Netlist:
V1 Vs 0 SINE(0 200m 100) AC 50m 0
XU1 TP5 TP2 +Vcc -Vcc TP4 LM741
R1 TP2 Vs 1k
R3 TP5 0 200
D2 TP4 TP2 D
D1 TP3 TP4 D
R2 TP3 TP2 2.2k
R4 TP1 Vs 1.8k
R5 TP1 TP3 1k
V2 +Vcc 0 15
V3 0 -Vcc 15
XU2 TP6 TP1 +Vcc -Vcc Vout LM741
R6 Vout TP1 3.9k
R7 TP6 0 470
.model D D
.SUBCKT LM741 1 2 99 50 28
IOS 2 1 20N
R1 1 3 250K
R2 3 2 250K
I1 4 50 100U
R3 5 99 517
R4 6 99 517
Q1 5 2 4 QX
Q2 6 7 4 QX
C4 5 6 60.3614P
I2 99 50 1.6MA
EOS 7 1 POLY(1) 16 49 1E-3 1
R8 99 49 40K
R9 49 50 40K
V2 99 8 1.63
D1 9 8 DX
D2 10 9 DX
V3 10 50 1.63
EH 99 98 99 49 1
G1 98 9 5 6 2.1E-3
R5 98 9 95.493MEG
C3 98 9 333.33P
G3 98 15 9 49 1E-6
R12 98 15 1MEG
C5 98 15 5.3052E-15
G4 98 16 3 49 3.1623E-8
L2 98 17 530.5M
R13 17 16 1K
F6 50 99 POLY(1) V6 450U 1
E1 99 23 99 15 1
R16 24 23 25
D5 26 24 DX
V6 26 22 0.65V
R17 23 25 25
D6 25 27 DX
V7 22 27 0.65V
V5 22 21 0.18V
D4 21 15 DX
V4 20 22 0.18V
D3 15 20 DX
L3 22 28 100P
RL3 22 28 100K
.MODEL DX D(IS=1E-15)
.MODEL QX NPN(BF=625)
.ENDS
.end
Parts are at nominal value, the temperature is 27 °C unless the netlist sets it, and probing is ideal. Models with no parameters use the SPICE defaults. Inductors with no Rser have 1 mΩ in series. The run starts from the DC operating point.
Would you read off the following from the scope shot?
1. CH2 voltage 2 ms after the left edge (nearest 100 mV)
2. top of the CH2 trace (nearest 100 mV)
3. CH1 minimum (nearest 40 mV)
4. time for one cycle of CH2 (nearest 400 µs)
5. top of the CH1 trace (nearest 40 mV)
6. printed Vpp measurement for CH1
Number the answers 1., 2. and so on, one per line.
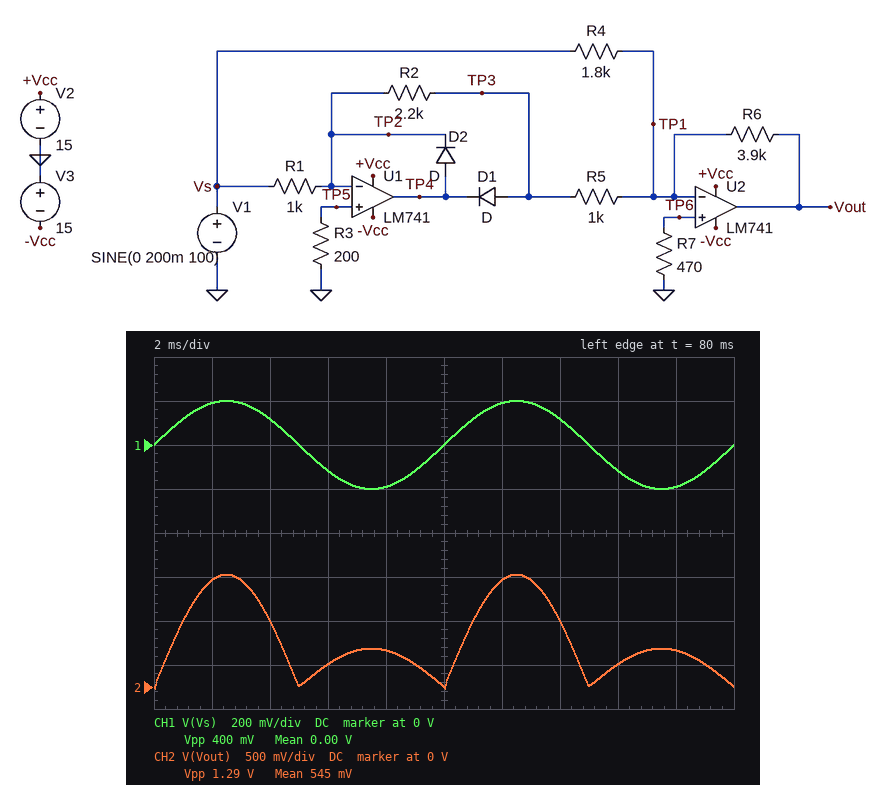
1. 1.2 V
2. 1.3 V
3. -200 mV
4. 10.0 ms
5. 200 mV
6. 400 mV
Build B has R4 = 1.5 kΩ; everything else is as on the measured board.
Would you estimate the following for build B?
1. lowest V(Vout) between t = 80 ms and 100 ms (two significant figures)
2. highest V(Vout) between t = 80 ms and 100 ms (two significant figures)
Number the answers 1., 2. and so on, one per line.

1. -22 mV
2. 1.2 V
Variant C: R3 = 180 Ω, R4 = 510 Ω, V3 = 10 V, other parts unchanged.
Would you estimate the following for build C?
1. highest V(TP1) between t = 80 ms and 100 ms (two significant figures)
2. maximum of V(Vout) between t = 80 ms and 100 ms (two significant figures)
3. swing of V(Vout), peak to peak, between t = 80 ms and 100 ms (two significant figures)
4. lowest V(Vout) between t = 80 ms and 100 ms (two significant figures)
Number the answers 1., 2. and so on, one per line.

1. 1.1 mV
2. 1.5 V
3. 1.6 V
4. -56 mV
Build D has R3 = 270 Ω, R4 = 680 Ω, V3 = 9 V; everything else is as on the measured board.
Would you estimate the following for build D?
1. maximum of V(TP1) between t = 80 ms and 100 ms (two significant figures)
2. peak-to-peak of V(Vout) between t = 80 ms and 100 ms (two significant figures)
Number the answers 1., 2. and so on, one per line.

1. 1.0 mV
2. 1.2 V
